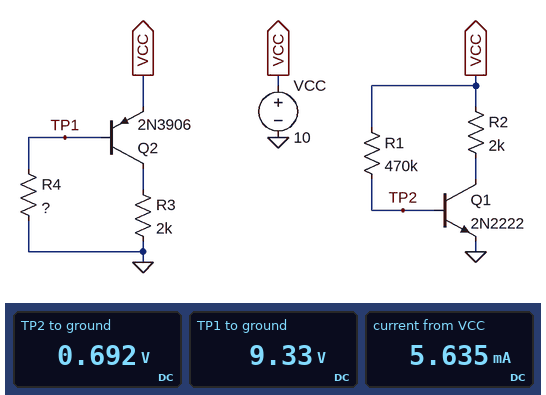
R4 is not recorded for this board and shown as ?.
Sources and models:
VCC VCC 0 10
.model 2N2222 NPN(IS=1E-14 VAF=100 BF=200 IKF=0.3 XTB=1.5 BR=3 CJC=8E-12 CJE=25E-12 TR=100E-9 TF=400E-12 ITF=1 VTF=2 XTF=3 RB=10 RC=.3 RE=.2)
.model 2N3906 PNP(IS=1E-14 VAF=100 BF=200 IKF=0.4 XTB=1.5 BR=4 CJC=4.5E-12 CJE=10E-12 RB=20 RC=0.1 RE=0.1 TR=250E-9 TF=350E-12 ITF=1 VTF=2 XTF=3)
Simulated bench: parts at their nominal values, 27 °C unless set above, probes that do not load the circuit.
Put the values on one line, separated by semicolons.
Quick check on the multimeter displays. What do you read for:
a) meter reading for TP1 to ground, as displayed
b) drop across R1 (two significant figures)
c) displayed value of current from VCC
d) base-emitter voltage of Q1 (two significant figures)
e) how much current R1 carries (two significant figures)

9.33 V; 9.3 V; 5.635 mA; 690 mV; 20 µA
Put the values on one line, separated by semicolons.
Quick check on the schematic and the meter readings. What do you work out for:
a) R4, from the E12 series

1.2 MΩ
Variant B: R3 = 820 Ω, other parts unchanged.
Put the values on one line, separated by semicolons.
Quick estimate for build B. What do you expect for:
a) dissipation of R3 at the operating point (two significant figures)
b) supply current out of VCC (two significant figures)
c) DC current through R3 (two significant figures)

2.3 mW; 5.7 mA; 1.7 mA
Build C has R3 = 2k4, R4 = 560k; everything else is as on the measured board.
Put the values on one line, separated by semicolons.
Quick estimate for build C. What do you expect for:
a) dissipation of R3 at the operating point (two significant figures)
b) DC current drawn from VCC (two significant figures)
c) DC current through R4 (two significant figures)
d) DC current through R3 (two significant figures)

27 mW; 7.3 mA; 17 µA; 3.3 mA
